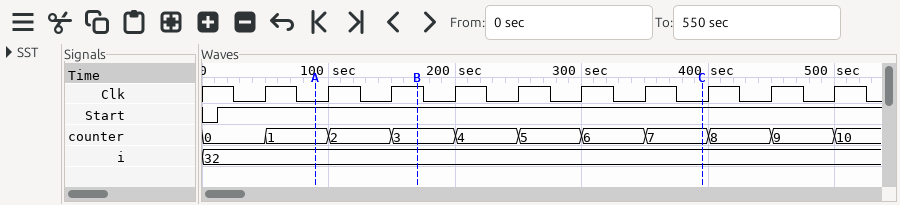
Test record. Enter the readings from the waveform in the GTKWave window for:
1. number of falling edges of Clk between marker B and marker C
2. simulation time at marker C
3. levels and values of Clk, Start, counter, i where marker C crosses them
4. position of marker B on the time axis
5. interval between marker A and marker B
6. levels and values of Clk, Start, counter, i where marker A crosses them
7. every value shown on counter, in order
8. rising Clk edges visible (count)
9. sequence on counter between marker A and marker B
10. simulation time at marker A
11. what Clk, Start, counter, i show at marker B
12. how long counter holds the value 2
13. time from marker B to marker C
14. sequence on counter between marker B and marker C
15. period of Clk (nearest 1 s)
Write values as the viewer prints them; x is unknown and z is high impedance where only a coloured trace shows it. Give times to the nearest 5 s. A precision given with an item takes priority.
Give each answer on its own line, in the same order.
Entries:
5
395 s
Clk=0, Start=1, counter=7, i=32
170 s
80 s
Clk=0, Start=1, counter=1, i=32
0, 1, 2, 3, 4, 5, 6, 7, 8, 9, 10
10
1, 2, 3
90 s
Clk=1, Start=1, counter=3, i=32
50 s
225 s
3, 4, 5, 6, 7
50 s
